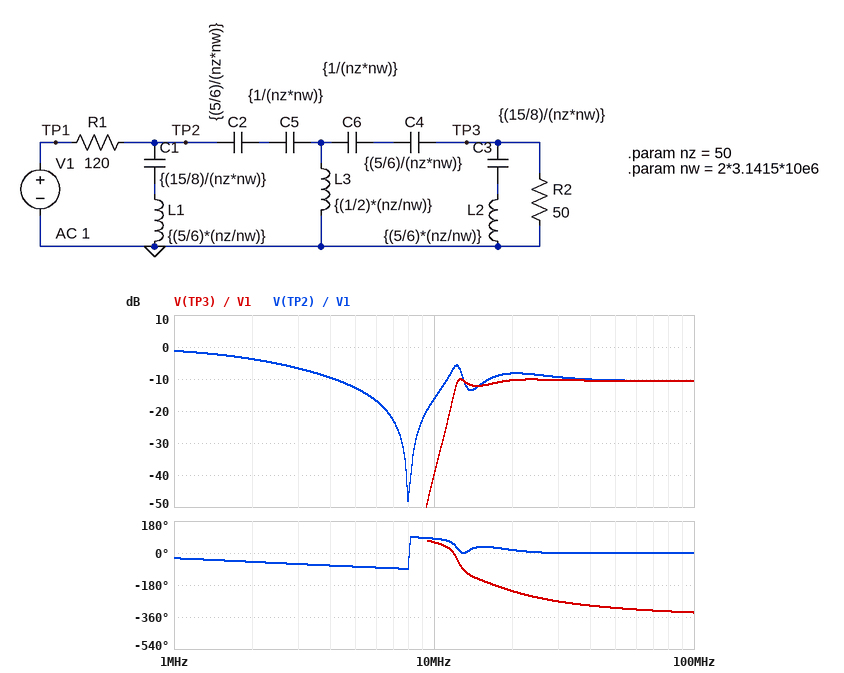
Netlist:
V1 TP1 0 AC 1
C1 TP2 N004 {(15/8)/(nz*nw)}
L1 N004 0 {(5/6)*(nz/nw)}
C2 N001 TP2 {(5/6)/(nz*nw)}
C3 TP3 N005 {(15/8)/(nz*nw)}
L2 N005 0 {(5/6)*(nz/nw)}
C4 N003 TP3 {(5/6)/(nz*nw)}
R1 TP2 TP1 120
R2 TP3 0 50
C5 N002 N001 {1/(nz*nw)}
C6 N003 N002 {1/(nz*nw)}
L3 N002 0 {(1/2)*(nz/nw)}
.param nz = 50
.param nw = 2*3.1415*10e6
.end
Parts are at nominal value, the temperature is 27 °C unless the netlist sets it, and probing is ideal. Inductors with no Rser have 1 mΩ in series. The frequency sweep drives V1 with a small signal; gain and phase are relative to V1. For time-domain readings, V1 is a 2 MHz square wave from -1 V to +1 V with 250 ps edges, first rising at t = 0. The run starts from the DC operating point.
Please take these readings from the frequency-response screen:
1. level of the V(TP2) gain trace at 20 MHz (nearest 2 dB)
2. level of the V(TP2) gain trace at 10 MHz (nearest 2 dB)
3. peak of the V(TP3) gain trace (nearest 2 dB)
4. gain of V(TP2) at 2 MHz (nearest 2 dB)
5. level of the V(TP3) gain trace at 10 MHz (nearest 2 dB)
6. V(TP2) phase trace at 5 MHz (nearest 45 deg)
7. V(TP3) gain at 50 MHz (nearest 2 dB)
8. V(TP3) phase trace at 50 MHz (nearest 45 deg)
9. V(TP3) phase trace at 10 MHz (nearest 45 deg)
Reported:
-8 dB
-16 dB
-10 dB
-4 dB
-40 dB
-90 deg
-10 dB
-315 deg
45 deg
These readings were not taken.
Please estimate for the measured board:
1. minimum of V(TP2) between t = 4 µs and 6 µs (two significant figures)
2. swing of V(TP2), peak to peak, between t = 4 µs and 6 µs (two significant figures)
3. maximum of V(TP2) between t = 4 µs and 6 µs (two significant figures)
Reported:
-900 mV
1.8 V
900 mV
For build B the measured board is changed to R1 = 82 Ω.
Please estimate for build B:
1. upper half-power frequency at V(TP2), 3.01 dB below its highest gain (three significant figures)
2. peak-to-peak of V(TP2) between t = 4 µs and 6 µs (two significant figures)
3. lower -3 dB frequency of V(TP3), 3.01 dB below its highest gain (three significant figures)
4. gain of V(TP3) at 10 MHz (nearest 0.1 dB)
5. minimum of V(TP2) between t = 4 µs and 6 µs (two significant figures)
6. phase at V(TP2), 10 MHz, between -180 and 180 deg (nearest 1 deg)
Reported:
2.42 MHz
2.0 V
12.1 MHz
-36.7 dB
-980 mV
77 deg
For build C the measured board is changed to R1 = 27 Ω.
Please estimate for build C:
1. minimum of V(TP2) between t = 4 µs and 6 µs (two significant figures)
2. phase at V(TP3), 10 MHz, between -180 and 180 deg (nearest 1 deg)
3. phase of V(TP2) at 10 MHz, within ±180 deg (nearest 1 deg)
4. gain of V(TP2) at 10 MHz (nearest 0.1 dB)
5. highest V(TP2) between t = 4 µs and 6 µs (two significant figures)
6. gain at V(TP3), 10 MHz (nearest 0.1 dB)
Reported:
-1.2 V
35 deg
55 deg
-4.9 dB
1.2 V
-28.5 dB
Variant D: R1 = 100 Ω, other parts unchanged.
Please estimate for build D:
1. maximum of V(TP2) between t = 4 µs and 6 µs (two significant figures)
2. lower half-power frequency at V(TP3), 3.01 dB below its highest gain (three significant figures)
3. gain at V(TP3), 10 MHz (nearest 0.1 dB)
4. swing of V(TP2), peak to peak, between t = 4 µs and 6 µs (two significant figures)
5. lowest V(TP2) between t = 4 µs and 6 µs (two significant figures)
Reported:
950 mV
12.1 MHz
-38.3 dB
1.9 V
-950 mV
